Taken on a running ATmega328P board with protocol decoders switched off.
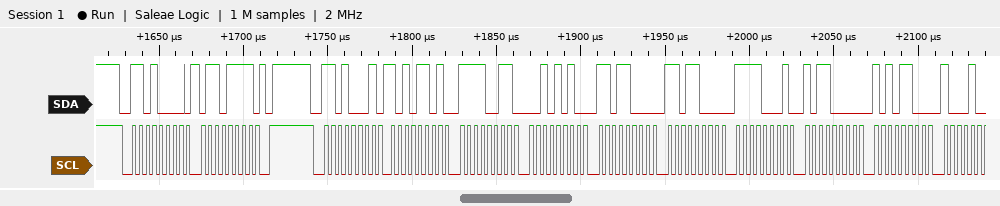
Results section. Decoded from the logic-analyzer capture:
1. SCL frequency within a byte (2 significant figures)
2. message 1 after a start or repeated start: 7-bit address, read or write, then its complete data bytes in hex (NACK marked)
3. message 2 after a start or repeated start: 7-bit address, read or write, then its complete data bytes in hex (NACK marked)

250 kHz
0x68 write: 6F
0x68 read: AD F3 2A D8 D8 F1 B0 AC
